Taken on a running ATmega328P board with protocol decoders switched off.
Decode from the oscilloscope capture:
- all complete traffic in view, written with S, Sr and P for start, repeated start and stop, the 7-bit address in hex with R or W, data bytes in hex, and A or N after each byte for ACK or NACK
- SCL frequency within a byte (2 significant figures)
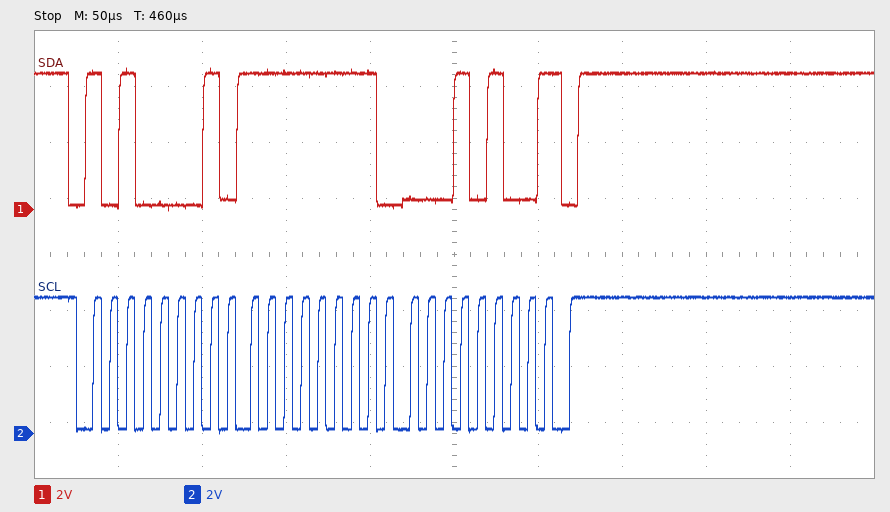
S 50R A FF A 14 N P
100 kHz
